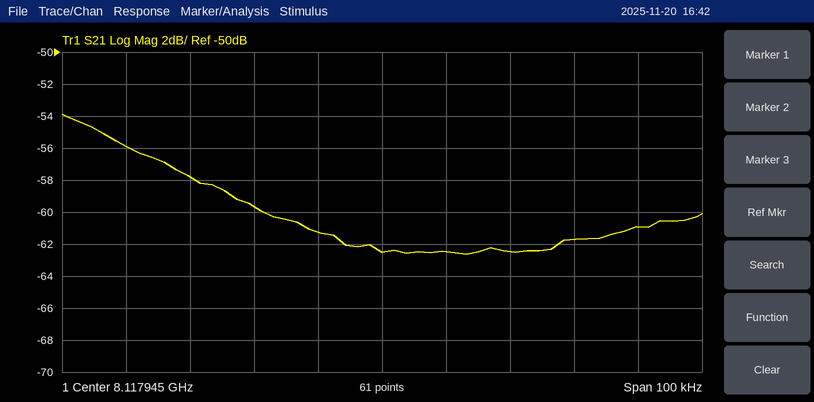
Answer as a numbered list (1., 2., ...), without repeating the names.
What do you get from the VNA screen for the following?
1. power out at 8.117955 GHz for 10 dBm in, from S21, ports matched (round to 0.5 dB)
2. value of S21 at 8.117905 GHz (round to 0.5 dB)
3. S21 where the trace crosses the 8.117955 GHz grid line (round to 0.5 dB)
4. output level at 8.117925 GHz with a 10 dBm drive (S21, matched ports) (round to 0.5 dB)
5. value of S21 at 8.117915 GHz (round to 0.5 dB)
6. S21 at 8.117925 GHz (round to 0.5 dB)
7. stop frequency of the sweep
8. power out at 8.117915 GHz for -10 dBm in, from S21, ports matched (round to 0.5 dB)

1. -52.5 dBm
2. -56.0 dB
3. -62.5 dB
4. -49.5 dBm
5. -58.0 dB
6. -59.5 dB
7. 8.117995 GHz
8. -68.0 dBm
